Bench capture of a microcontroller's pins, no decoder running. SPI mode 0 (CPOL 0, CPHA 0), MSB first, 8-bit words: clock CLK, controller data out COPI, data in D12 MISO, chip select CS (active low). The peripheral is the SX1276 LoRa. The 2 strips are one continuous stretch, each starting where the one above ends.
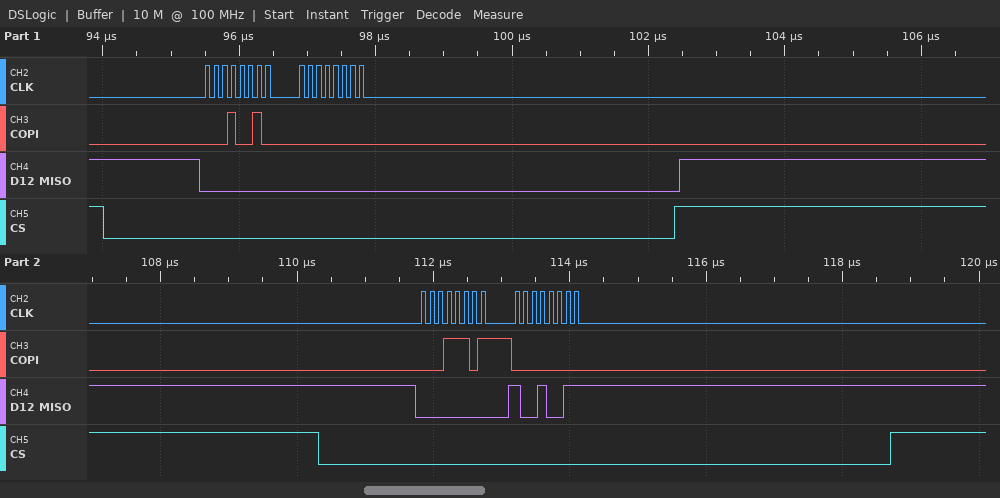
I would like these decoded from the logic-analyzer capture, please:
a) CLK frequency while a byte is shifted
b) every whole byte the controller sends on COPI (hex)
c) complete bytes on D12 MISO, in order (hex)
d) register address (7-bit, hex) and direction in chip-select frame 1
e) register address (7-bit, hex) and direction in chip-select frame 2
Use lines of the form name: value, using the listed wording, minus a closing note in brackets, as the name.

CLK frequency while a byte is shifted: 8 MHz
every whole byte the controller sends on COPI: 12 00 1D 00
complete bytes on D12 MISO, in order: 00 00 00 93
register address (7-bit, hex) and direction in chip-select frame 1: 0x12 read
register address (7-bit, hex) and direction in chip-select frame 2: 0x1D read
